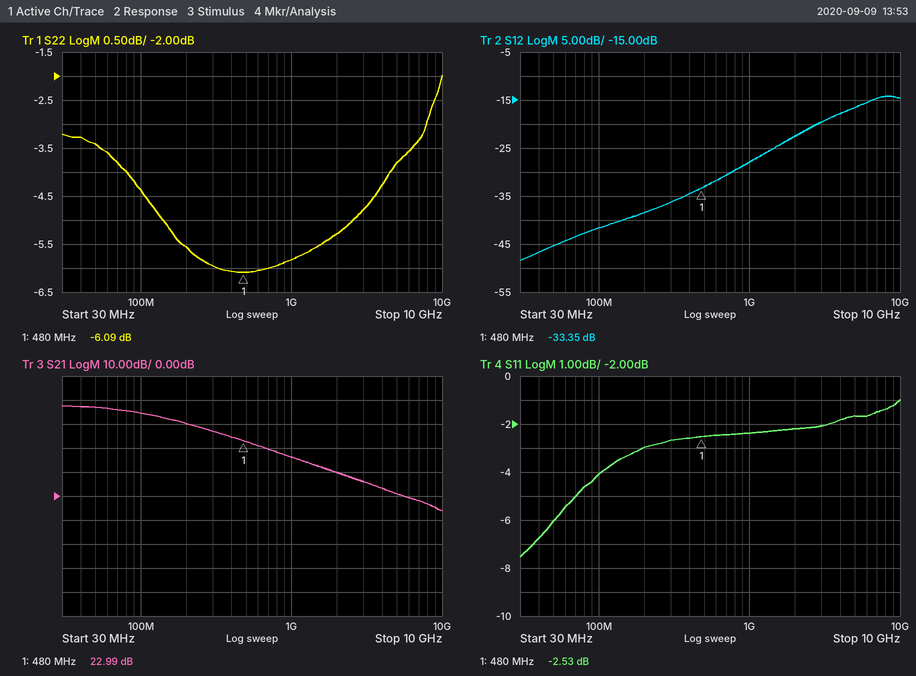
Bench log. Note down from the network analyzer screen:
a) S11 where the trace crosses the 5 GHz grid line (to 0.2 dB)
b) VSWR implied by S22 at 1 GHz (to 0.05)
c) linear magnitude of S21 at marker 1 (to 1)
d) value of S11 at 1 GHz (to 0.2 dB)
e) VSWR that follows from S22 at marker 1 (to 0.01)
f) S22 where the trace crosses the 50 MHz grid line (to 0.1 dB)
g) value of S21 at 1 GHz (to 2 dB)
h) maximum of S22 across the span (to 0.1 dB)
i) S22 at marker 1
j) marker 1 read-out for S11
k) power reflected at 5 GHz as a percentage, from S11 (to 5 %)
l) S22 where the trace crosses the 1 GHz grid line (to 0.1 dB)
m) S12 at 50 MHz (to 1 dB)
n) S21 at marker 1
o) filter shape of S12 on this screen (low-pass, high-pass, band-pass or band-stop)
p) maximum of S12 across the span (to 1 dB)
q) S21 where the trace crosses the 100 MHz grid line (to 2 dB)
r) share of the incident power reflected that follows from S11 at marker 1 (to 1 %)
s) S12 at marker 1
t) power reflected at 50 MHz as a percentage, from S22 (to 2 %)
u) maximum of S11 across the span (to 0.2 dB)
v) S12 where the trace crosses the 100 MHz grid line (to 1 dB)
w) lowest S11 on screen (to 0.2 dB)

-1.6 dB
3.10
14
-2.4 dB
2.97
-3.4 dB
16 dB
-2.0 dB
-6.09 dB
-2.53 dB
70 %
-5.8 dB
-45 dB
22.99 dB
high-pass
-14 dB
34 dB
56 %
-33.35 dB
46 %
-1.0 dB
-42 dB
-7.6 dB
